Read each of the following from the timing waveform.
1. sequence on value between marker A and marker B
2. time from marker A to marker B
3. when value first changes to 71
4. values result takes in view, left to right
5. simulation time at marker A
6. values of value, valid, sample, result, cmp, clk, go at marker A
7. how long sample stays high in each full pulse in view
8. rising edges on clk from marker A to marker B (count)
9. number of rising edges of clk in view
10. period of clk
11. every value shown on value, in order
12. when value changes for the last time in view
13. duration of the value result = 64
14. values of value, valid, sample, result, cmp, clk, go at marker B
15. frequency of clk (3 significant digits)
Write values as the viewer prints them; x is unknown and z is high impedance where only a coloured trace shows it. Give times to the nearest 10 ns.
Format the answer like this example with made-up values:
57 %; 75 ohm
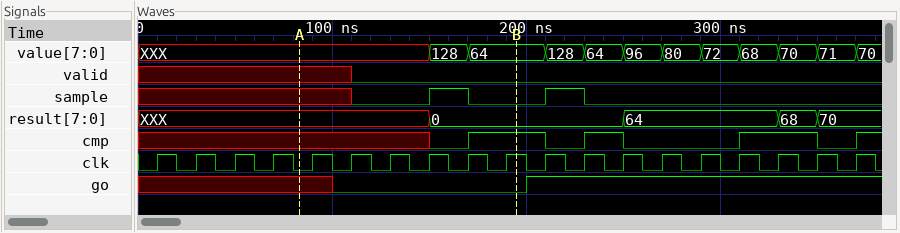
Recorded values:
XXX, 128, 64; 110 ns; 350 ns; XXX, 0, 64, 68, 70; 80 ns; value=XXX, valid=x, sample=x, result=XXX, cmp=x, clk=0, go=x; 20 ns, 20 ns; 6; 19; 20 ns; XXX, 128, 64, 128, 64, 96, 80, 72, 68, 70, 71, 70; 370 ns; 80 ns; value=64, valid=0, sample=0, result=0, cmp=1, clk=1, go=0; 50.0 MHz
